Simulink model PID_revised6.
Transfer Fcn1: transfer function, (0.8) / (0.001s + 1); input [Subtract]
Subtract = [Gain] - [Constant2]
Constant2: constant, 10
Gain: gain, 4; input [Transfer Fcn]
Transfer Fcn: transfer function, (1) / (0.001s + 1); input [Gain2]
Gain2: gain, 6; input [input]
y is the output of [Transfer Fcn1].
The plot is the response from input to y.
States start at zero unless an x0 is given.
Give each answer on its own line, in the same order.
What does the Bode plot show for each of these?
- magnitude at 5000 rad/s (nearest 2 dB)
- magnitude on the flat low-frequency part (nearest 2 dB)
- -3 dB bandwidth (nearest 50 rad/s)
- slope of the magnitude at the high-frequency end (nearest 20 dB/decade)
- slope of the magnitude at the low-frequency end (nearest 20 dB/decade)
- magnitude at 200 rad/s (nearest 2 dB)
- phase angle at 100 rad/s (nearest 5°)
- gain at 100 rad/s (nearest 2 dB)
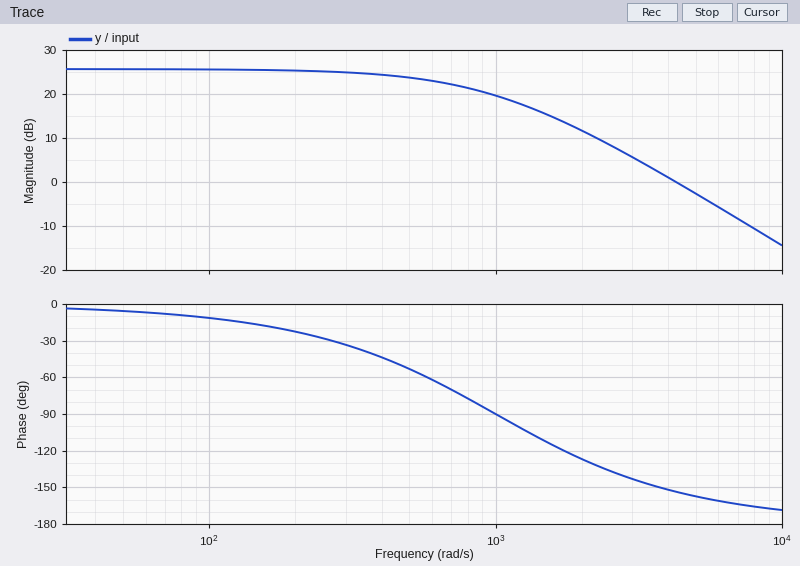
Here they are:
-2 dB
26 dB
650 rad/s
-40 dB/decade
0 dB/decade
26 dB
-10°
26 dB
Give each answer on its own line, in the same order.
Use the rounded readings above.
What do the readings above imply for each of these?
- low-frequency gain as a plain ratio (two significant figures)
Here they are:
20
